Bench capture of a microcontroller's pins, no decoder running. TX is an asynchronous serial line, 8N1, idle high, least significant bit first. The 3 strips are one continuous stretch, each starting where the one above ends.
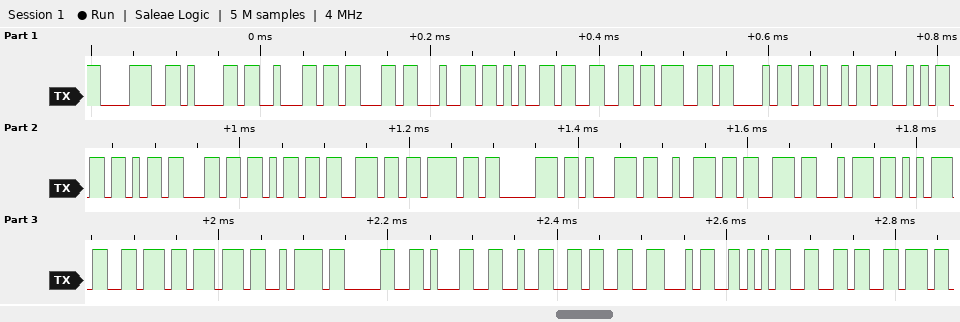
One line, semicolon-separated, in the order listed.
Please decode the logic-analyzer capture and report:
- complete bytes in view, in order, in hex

0x38 0x61 0x62 0x63 0x64 0x65 0x66 0x67 0x68 0x69 0x6A 0x6B 0x6C 0x6D 0x6E 0x6F 0x70 0x71 0x72 0x73 0x74 0x75 0x76 0x77 0x7A 0x30 0x31 0x32 0x33 0x34 0x35 0x36
